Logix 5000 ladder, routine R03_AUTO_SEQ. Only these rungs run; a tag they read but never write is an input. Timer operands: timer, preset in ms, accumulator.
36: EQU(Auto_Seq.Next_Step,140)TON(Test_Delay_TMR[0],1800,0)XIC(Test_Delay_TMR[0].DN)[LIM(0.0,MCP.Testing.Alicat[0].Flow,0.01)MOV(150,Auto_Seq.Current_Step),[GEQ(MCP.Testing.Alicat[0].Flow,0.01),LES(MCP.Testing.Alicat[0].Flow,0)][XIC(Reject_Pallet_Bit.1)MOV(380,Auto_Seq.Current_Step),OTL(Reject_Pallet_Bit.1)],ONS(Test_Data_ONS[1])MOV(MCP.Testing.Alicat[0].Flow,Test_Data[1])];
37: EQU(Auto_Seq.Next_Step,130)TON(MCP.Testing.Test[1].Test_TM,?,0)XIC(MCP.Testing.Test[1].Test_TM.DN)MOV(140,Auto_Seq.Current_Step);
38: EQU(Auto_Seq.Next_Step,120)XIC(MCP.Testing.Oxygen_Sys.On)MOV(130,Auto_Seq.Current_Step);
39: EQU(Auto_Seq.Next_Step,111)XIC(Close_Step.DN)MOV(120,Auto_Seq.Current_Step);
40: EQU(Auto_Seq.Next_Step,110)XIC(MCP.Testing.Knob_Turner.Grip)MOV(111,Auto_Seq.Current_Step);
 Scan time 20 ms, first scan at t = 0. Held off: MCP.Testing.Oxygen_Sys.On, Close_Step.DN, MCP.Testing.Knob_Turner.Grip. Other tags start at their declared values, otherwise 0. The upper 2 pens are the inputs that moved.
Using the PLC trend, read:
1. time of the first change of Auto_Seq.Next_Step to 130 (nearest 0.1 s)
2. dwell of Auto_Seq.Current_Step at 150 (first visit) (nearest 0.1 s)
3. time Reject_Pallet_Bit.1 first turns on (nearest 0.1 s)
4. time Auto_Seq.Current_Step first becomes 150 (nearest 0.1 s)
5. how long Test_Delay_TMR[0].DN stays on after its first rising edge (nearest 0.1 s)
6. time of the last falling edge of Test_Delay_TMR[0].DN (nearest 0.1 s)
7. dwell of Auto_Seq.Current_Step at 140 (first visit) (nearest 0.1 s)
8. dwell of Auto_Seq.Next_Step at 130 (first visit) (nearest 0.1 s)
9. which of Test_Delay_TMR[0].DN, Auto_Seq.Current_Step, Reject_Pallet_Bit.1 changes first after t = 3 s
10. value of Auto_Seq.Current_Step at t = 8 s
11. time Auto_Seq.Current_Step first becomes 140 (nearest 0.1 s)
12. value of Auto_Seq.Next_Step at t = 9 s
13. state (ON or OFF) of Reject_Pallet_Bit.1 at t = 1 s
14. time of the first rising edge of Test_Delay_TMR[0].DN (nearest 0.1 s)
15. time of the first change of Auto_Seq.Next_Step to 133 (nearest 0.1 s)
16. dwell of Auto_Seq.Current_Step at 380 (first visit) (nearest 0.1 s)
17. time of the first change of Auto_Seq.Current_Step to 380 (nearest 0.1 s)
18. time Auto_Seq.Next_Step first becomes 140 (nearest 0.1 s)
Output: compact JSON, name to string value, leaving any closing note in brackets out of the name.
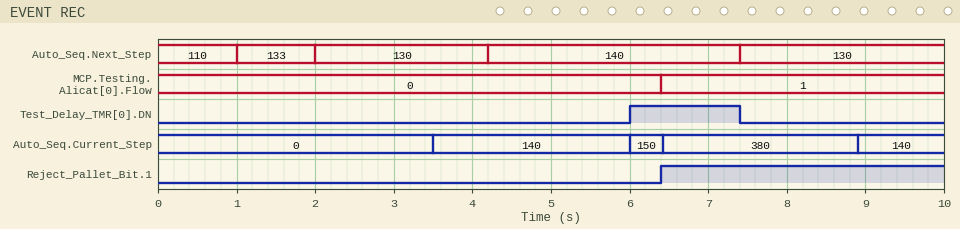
{"time of the first change of Auto_Seq.Next_Step to 130": "2.0 s", "dwell of Auto_Seq.Current_Step at 150 (first visit)": "0.4 s", "time Reject_Pallet_Bit.1 first turns on": "6.4 s", "time Auto_Seq.Current_Step first becomes 150": "6.0 s", "how long Test_Delay_TMR[0].DN stays on after its first rising edge": "1.4 s", "time of the last falling edge of Test_Delay_TMR[0].DN": "7.4 s", "dwell of Auto_Seq.Current_Step at 140 (first visit)": "2.5 s", "dwell of Auto_Seq.Next_Step at 130 (first visit)": "2.2 s", "which of Test_Delay_TMR[0].DN, Auto_Seq.Current_Step, Reject_Pallet_Bit.1 changes first after t = 3 s": "Auto_Seq.Current_Step", "value of Auto_Seq.Current_Step at t = 8 s": "380", "time Auto_Seq.Current_Step first becomes 140": "3.5 s", "value of Auto_Seq.Next_Step at t = 9 s": "130", "state (ON or OFF) of Reject_Pallet_Bit.1 at t = 1 s": "OFF", "time of the first rising edge of Test_Delay_TMR[0].DN": "6.0 s", "time of the first change of Auto_Seq.Next_Step to 133": "1.0 s", "dwell of Auto_Seq.Current_Step at 380 (first visit)": "2.5 s", "time of the first change of Auto_Seq.Current_Step to 380": "6.4 s", "time Auto_Seq.Next_Step first becomes 140": "4.2 s"}
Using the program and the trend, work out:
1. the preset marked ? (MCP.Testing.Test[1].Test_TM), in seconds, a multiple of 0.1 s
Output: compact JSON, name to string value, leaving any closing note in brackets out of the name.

{"the preset marked ? (MCP.Testing.Test[1].Test_TM), in seconds, a multiple of 0.1 s": "1.5 s"}
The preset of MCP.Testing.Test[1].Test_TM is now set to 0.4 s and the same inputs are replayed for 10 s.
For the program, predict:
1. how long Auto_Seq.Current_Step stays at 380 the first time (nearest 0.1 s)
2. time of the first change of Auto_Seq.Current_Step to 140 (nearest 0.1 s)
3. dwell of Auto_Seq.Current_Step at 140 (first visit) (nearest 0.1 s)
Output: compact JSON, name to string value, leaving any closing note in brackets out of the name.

{"how long Auto_Seq.Current_Step stays at 380 the first time": "1.4 s", "time of the first change of Auto_Seq.Current_Step to 140": "2.4 s", "dwell of Auto_Seq.Current_Step at 140 (first visit)": "3.6 s"}
